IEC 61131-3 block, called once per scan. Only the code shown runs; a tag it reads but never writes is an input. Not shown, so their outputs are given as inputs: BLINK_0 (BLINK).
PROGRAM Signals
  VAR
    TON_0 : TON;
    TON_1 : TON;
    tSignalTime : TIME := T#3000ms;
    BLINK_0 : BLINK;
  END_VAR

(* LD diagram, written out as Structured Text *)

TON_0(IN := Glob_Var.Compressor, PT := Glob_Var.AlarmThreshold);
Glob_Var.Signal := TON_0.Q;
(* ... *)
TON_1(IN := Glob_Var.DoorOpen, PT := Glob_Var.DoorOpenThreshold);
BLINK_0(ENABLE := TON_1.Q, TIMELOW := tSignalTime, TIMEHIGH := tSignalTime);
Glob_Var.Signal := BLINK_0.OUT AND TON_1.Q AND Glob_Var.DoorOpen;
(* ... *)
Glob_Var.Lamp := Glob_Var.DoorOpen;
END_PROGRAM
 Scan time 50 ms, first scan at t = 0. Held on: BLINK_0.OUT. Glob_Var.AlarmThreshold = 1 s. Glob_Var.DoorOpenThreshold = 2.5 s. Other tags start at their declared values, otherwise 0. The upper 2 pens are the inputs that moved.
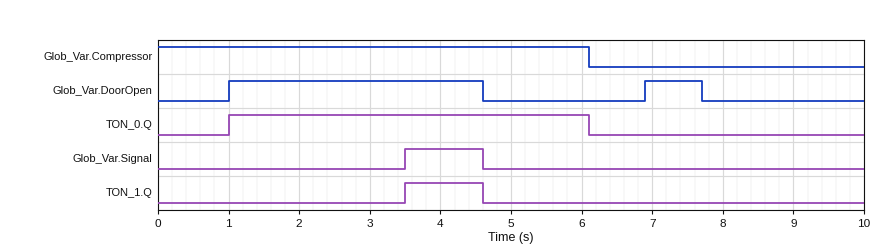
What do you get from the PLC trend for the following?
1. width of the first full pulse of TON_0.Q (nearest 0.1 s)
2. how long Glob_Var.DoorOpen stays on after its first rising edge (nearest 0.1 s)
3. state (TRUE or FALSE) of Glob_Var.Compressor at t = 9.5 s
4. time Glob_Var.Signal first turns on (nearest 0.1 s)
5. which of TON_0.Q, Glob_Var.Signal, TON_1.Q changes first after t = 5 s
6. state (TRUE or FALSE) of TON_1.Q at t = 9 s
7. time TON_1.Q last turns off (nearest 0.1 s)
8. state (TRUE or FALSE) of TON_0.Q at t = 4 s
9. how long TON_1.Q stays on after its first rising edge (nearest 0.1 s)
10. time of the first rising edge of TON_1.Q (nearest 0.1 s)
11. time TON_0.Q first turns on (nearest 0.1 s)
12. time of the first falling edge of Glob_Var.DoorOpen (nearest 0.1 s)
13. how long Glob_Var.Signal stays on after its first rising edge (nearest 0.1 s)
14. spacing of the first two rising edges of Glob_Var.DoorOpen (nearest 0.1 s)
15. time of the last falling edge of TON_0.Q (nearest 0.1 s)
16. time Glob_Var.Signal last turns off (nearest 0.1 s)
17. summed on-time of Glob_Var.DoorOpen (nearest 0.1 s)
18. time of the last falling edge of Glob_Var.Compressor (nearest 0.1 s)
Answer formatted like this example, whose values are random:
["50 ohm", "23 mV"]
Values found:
["5.1 s", "3.6 s", "FALSE", "3.5 s", "TON_0.Q", "FALSE", "4.6 s", "TRUE", "1.1 s", "3.5 s", "1.0 s", "4.6 s", "1.1 s", "5.9 s", "6.1 s", "4.6 s", "4.4 s", "6.1 s"]
